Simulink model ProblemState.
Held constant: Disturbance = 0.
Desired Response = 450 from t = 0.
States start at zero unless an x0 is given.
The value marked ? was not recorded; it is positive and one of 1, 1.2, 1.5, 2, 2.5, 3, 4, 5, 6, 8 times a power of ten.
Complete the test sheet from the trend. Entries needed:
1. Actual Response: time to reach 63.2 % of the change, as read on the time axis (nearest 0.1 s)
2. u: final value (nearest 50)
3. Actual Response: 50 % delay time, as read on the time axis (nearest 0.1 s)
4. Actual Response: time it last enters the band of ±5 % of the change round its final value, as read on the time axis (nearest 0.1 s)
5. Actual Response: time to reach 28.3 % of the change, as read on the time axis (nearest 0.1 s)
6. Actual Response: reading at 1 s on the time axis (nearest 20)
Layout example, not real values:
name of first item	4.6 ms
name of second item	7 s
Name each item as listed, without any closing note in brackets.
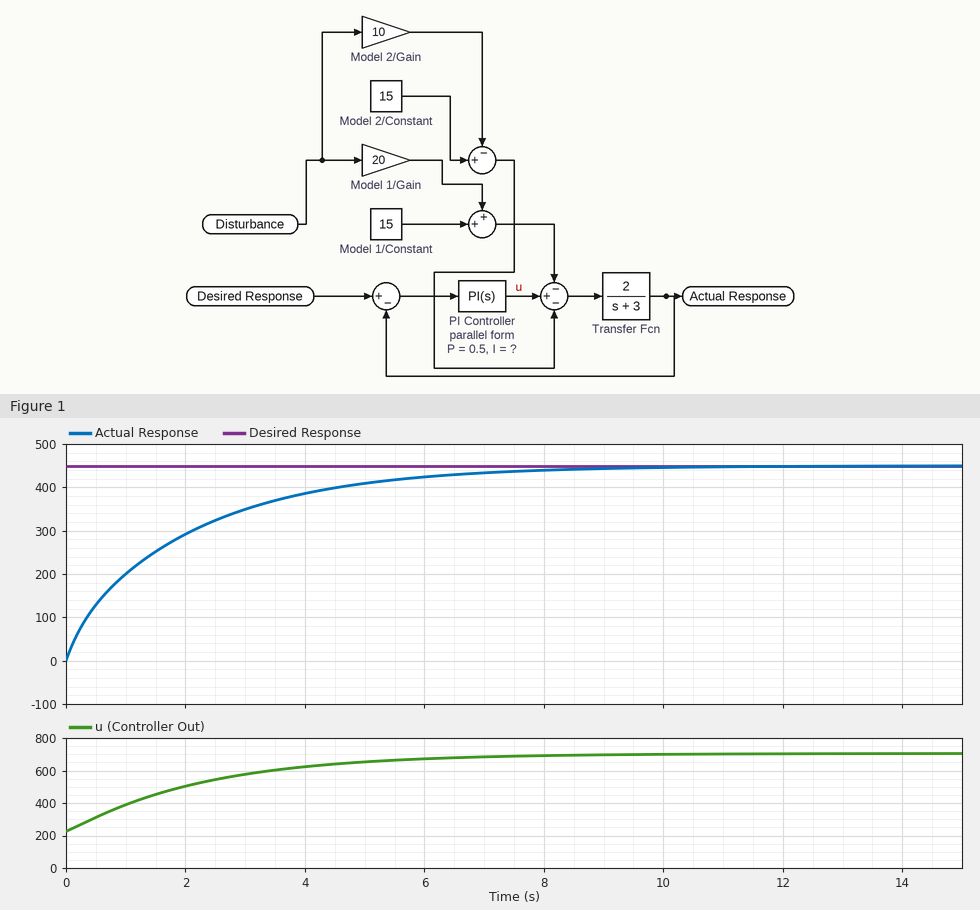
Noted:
Actual Response: time to reach 63.2 % of the change, as read on the time axis	1.9 s
u: final value	700
Actual Response: 50 % delay time, as read on the time axis	1.2 s
Actual Response: time it last enters the band of ±5 % of the change round its final value, as read on the time axis	6.3 s
Actual Response: time to reach 28.3 % of the change, as read on the time axis	0.5 s
Actual Response: reading at 1 s on the time axis	200
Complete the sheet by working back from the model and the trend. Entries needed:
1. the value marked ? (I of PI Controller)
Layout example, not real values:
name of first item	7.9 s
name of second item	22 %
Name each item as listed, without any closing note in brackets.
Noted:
the value marked ?	0.8
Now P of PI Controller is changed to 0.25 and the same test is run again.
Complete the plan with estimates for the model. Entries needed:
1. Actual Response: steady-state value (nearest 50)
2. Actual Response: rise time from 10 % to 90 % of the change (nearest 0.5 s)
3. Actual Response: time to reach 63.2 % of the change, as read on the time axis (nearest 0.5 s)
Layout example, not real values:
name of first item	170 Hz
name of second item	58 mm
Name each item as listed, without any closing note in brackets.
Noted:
Actual Response: steady-state value	450
Actual Response: rise time from 10 % to 90 % of the change	4.0 s
Actual Response: time to reach 63.2 % of the change, as read on the time axis	2.0 s
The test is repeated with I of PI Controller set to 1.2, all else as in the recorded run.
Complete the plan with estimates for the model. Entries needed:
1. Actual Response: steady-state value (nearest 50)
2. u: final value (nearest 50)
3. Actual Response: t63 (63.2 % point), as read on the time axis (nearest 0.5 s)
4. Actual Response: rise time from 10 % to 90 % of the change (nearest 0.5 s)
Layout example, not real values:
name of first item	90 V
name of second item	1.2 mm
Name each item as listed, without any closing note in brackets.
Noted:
Actual Response: steady-state value	450
u: final value	700
Actual Response: t63 (63.2 % point), as read on the time axis	1.5 s
Actual Response: rise time from 10 % to 90 % of the change	3.0 s
